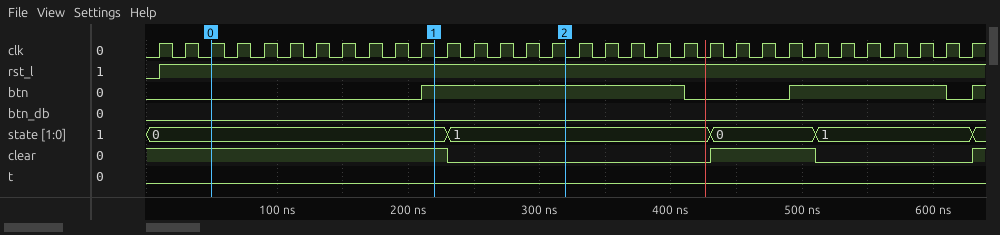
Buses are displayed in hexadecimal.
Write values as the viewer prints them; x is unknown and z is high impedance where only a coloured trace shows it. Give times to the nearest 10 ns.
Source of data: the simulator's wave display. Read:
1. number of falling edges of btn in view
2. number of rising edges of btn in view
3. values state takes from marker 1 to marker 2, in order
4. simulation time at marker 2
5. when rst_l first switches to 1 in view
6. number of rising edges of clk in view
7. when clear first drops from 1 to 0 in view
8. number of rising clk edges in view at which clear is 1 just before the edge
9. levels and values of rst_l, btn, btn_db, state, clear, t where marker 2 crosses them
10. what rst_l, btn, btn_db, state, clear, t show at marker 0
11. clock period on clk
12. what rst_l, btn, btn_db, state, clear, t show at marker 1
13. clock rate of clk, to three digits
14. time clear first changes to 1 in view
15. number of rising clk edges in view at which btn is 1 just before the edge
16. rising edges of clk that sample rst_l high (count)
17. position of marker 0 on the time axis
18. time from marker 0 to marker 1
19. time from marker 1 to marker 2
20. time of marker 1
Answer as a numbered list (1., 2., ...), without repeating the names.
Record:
1. 2
2. 3
3. 0, 1
4. 320 ns
5. 10 ns
6. 32
7. 230 ns
8. 16
9. rst_l=1, btn=1, btn_db=0, state=1, clear=0, t=0
10. rst_l=1, btn=0, btn_db=0, state=0, clear=1, t=0
11. 20 ns
12. rst_l=1, btn=1, btn_db=0, state=0, clear=1, t=0
13. 50.0 MHz
14. 430 ns
15. 16
16. 31
17. 50 ns
18. 170 ns
19. 100 ns
20. 220 ns
